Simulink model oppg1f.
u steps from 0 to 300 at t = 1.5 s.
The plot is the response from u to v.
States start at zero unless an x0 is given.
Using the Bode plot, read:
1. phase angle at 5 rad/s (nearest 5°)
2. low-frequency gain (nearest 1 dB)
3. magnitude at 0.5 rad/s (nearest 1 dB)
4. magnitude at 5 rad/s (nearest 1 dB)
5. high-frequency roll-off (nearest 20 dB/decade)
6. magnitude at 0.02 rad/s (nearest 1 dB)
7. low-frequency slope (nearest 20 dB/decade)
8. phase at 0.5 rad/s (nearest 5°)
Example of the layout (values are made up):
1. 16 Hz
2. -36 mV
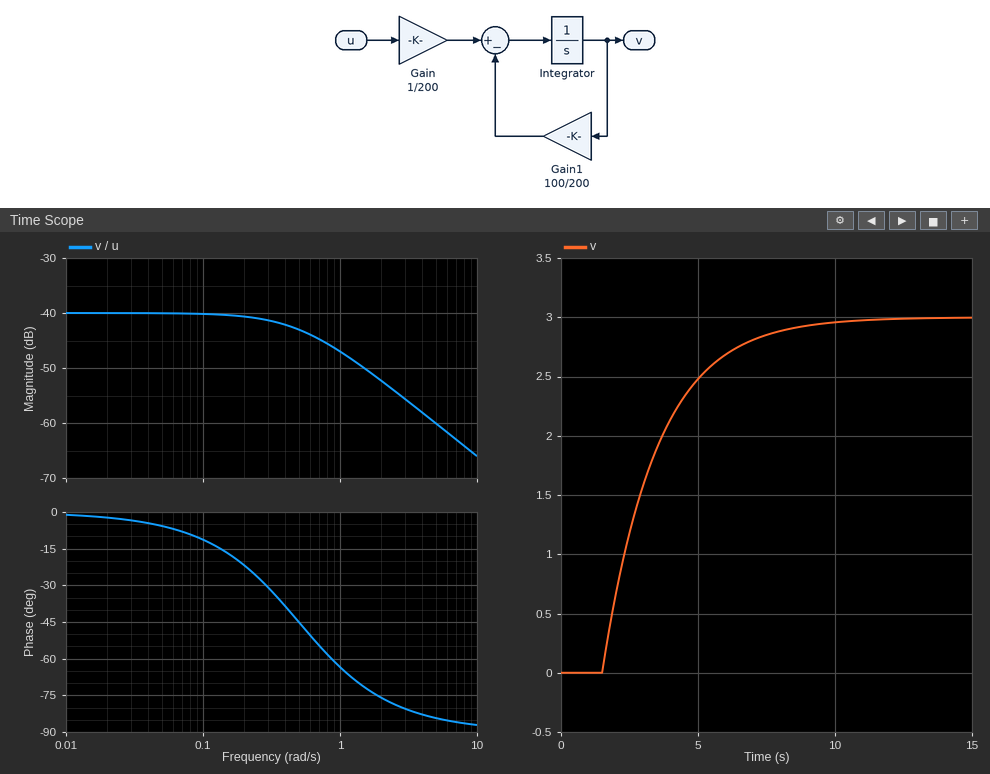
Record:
1. -85°
2. -40 dB
3. -43 dB
4. -60 dB
5. -20 dB/decade
6. -40 dB
7. 0 dB/decade
8. -45°
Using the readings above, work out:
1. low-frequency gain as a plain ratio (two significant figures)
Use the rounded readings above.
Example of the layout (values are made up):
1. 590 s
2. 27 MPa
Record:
1. 0.010
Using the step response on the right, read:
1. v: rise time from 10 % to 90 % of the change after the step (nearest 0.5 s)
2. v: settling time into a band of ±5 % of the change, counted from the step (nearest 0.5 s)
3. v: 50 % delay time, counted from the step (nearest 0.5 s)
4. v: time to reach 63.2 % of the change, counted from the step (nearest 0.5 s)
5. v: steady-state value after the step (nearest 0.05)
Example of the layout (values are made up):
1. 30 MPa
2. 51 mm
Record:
1. 4.5 s
2. 6.0 s
3. 1.5 s
4. 2.0 s
5. 3.00
